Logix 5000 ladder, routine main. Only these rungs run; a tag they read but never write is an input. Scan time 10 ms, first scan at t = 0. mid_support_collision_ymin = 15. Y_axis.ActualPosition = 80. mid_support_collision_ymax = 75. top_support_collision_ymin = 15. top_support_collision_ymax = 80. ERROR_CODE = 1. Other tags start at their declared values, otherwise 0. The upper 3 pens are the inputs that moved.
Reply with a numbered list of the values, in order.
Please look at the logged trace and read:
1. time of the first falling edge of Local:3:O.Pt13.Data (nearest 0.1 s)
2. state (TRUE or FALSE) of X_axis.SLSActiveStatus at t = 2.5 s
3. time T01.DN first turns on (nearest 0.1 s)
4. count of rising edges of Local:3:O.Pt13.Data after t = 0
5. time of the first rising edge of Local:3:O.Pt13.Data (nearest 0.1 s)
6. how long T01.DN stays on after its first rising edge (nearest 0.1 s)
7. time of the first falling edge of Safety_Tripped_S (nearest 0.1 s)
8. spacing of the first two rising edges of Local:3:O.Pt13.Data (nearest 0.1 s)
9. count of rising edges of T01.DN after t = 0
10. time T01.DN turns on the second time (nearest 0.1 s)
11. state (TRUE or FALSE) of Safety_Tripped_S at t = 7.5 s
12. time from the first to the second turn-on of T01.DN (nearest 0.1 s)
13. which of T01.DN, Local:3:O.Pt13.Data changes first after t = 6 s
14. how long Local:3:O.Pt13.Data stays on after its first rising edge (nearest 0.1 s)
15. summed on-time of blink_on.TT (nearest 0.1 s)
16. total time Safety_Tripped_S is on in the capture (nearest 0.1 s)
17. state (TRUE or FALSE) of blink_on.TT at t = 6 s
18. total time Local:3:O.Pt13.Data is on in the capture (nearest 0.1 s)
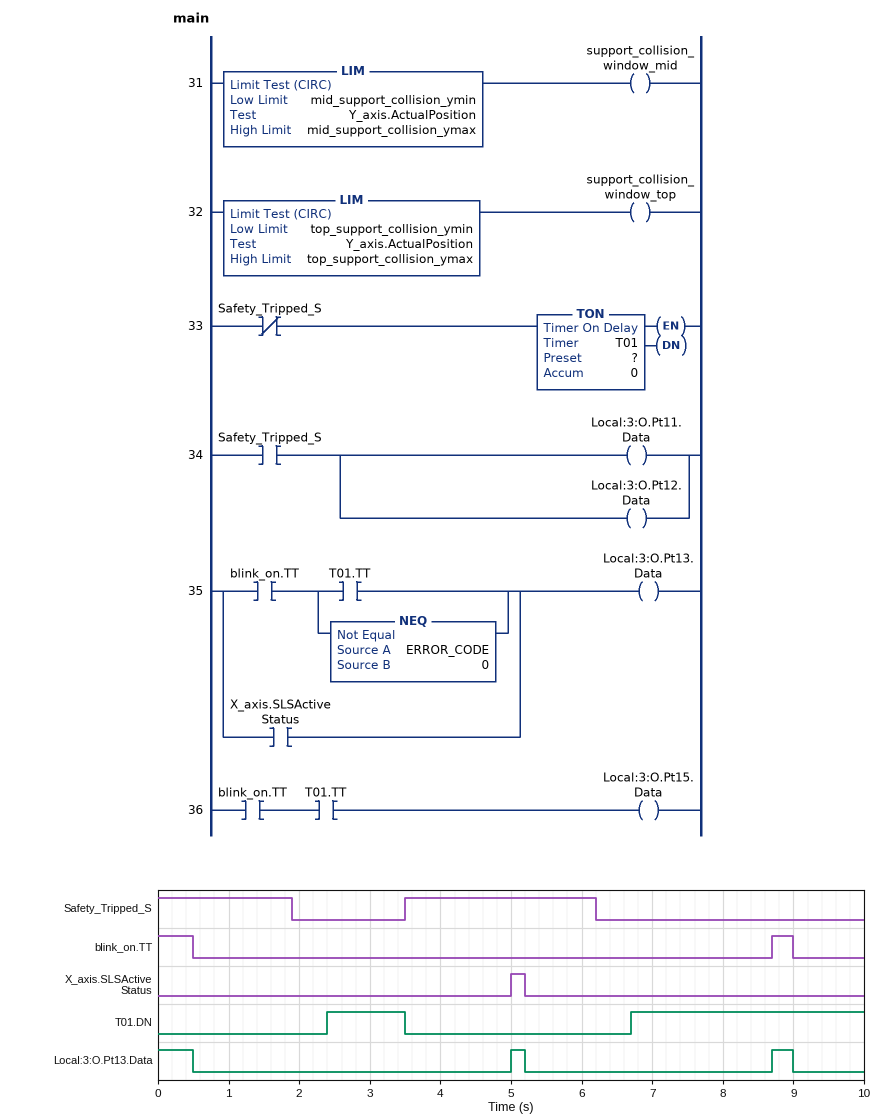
1. 0.5 s
2. FALSE
3. 2.4 s
4. 2
5. 5.0 s
6. 1.1 s
7. 1.9 s
8. 3.7 s
9. 2
10. 6.7 s
11. FALSE
12. 4.3 s
13. T01.DN
14. 0.2 s
15. 0.8 s
16. 4.6 s
17. FALSE
18. 1.0 s
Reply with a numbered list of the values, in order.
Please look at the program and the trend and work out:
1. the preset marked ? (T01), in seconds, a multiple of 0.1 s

1. 0.5 s
